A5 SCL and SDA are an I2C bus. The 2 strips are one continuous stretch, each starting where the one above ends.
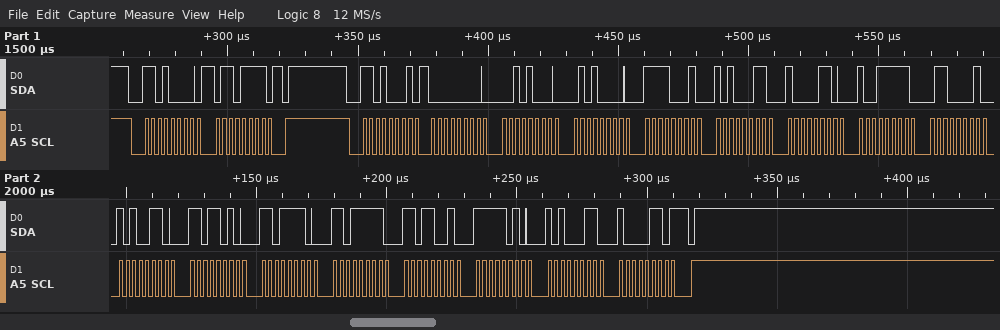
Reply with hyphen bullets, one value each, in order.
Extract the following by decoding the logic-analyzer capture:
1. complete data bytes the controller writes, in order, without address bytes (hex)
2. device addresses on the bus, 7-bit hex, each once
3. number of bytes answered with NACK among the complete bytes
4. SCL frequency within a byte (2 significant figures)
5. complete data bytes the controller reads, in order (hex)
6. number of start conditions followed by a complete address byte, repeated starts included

- 6F
- 0x68
- 1
- 400 kHz
- 00 28 50 F1 A3 86 9F 61 A6 DA DE DF D9 FA A3 86
- 2
